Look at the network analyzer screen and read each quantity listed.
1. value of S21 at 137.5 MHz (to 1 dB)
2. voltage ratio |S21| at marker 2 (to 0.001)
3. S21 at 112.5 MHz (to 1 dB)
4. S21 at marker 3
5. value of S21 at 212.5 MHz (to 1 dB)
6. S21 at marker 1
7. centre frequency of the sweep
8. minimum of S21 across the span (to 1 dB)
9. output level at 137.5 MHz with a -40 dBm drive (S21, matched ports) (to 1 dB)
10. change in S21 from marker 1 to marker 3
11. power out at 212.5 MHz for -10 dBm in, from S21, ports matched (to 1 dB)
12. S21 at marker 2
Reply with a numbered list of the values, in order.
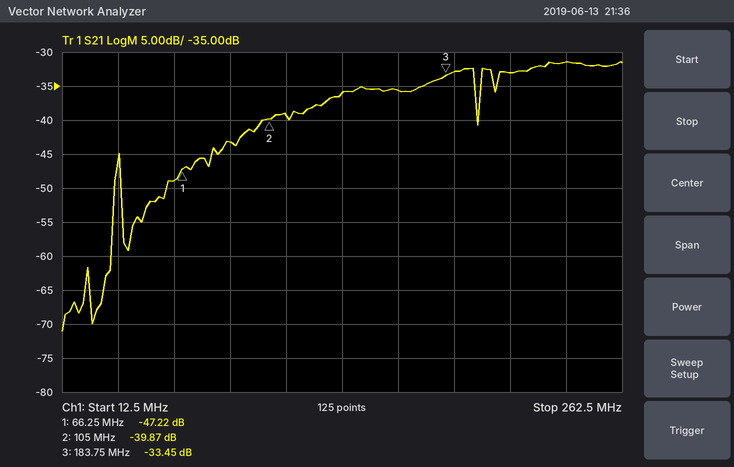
1. -36 dB
2. 0.010
3. -39 dB
4. -33.45 dB
5. -33 dB
6. -47.22 dB
7. 137.5 MHz
8. -71 dB
9. -76 dBm
10. 13.77 dB
11. -43 dBm
12. -39.87 dB
